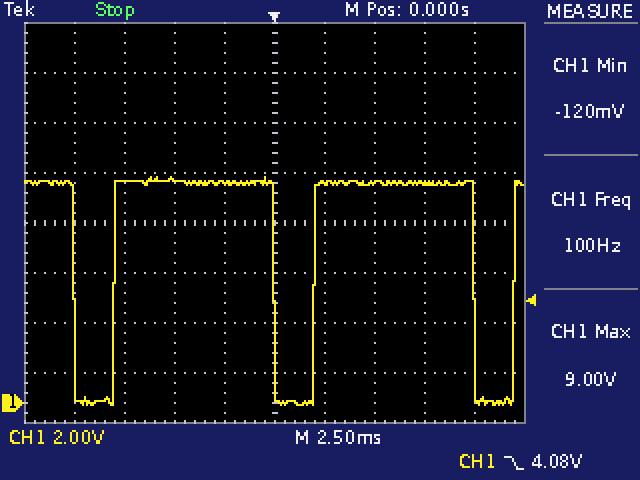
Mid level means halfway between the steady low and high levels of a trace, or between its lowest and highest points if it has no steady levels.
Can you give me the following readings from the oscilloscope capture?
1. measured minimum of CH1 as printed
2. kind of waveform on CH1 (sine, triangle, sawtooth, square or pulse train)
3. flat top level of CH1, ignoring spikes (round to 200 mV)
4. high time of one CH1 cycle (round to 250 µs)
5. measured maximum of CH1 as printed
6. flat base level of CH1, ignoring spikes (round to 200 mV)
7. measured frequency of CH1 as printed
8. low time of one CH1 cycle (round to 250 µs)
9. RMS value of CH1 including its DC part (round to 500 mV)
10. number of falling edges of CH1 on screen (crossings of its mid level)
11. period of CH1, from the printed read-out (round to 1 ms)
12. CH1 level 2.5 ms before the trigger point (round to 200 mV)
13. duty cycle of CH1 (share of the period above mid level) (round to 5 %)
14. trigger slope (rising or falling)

-120 mV
pulse train
8.8 V
8.00 ms
9.00 V
0.0 V
100 Hz
2.00 ms
8.0 V
3
10 ms
8.8 V
80 %
falling
